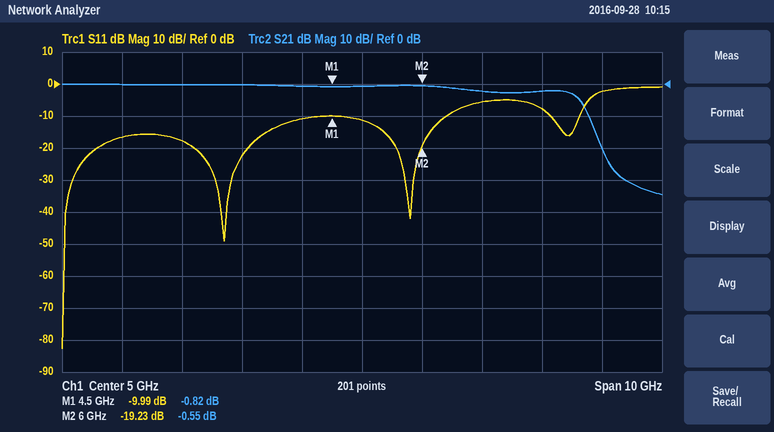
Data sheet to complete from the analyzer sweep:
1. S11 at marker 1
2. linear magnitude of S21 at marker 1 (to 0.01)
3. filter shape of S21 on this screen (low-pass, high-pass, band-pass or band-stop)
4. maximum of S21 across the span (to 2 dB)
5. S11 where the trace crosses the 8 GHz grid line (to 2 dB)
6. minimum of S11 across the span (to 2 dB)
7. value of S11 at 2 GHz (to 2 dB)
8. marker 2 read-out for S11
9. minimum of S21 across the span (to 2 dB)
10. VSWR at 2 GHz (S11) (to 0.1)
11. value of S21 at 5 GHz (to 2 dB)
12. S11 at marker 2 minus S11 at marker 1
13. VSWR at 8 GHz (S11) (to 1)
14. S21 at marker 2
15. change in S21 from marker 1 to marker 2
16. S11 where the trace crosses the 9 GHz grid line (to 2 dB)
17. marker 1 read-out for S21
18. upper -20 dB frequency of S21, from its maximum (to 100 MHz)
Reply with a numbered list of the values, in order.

1. -9.99 dB
2. 0.91
3. low-pass
4. 0 dB
5. -8 dB
6. -82 dB
7. -18 dB
8. -19.23 dB
9. -34 dB
10. 1.3
11. 0 dB
12. -9.24 dB
13. 2
14. -0.55 dB
15. 0.27 dB
16. -2 dB
17. -0.82 dB
18. 9.0 GHz
